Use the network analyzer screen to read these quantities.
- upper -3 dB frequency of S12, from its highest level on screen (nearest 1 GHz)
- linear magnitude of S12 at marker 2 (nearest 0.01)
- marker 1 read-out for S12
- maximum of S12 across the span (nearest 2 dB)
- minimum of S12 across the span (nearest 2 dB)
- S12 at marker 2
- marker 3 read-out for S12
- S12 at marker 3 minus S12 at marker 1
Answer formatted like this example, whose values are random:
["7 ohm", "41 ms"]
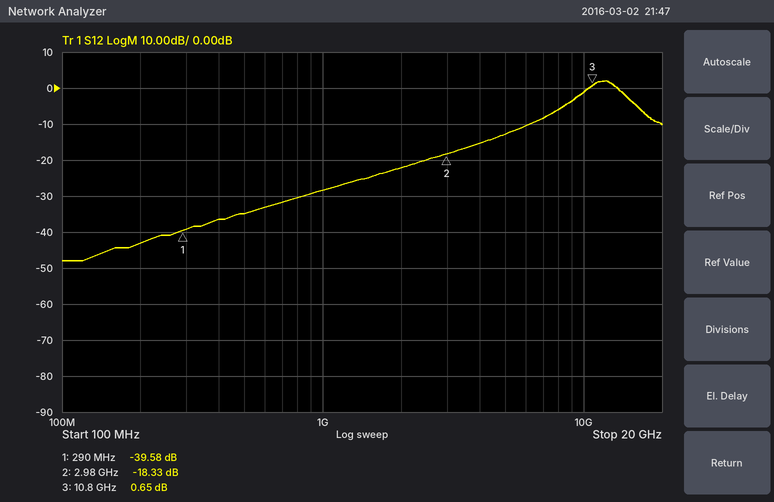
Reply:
["14 GHz", "0.12", "-39.58 dB", "2 dB", "-48 dB", "-18.33 dB", "0.65 dB", "40.23 dB"]
